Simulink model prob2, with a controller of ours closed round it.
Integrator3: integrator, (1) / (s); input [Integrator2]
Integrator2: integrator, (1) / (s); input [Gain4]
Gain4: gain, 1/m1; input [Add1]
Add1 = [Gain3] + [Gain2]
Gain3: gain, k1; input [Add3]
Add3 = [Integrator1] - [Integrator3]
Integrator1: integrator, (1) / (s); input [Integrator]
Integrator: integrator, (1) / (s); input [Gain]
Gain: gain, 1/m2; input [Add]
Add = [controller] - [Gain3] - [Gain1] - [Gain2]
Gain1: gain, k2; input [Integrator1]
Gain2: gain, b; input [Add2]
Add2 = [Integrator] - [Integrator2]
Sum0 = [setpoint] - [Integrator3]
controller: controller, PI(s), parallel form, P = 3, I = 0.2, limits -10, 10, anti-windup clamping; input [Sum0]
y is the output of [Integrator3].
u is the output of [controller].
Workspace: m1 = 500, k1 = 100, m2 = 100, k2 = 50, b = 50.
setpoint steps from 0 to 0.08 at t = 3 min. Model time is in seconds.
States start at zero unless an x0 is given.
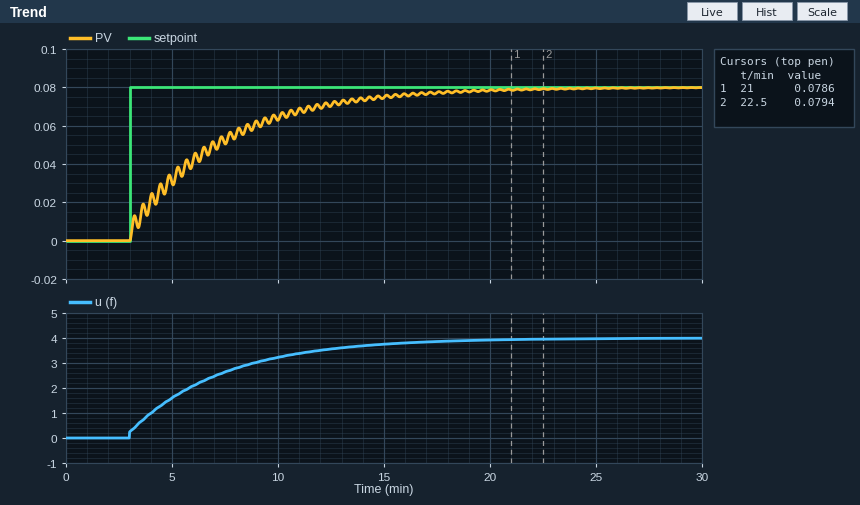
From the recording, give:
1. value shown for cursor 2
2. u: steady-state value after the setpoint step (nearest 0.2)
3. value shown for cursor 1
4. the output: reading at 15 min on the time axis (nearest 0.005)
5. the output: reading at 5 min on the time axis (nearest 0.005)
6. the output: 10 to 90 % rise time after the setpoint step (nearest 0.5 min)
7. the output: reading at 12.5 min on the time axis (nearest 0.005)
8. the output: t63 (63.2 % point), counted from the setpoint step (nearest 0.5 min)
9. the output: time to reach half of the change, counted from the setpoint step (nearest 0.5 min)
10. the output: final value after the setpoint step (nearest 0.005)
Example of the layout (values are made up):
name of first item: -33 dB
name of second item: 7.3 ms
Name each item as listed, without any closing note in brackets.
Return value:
value shown for cursor 2: 0.0794
u: steady-state value after the setpoint step: 4.0
value shown for cursor 1: 0.0786
the output: reading at 15 min on the time axis: 0.075
the output: reading at 5 min on the time axis: 0.030
the output: 10 to 90 % rise time after the setpoint step: 9.5 min
the output: reading at 12.5 min on the time axis: 0.070
the output: t63 (63.2 % point), counted from the setpoint step: 4.0 min
the output: time to reach half of the change, counted from the setpoint step: 2.5 min
the output: final value after the setpoint step: 0.080
